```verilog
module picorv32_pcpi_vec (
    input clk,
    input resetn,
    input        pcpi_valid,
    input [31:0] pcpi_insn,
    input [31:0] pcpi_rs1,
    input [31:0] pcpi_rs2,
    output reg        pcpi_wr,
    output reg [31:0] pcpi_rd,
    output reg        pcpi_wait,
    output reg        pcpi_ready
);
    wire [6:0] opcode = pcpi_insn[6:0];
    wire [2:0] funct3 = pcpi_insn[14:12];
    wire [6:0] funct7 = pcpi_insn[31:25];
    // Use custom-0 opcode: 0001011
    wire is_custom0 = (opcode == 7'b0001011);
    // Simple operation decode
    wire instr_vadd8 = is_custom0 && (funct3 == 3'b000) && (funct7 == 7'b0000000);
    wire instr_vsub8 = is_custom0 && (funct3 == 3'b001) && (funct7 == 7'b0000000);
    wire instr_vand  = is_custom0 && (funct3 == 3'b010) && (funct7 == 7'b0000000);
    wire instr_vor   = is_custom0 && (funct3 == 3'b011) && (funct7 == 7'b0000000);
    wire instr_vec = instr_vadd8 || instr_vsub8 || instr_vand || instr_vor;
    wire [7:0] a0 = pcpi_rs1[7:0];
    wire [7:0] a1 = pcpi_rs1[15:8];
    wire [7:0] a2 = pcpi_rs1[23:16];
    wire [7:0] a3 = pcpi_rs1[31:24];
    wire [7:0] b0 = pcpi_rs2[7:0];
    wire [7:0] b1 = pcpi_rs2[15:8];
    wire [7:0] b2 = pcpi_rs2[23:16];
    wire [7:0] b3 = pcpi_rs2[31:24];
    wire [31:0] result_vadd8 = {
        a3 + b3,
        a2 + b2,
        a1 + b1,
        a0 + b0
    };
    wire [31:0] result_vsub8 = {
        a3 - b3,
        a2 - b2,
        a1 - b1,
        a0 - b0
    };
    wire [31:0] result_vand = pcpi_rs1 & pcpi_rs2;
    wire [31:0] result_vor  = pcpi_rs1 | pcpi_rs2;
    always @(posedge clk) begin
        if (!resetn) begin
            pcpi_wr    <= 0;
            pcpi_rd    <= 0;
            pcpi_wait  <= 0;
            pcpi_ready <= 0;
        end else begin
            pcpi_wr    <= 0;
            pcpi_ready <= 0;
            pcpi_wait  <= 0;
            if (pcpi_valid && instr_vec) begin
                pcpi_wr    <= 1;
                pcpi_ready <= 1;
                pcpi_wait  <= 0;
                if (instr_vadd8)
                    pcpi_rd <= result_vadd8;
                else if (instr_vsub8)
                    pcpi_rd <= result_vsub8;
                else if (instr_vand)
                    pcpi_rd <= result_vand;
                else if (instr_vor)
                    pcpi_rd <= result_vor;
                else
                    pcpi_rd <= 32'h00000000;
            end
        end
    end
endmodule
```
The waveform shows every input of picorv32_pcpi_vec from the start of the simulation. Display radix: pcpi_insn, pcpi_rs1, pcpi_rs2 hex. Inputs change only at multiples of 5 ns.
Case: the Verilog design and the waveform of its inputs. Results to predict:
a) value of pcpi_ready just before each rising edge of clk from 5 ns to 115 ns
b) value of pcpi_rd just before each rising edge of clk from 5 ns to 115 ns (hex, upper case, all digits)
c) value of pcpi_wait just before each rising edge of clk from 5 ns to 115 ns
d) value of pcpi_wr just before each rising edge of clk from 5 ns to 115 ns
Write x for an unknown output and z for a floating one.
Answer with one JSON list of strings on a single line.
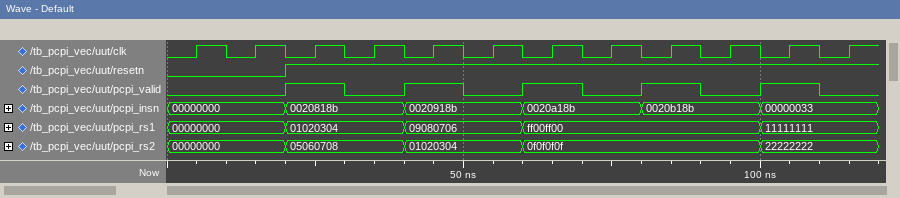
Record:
["x 0 0 1 0 1 0 1 0 1 0 0", "x, 00000000, 00000000, 06080A0C, 06080A0C, 08060402, 08060402, 0F000F00, 0F000F00, FF0FFF0F, FF0FFF0F, FF0FFF0F", "x 0 0 0 0 0 0 0 0 0 0 0", "x 0 0 1 0 1 0 1 0 1 0 0"]
